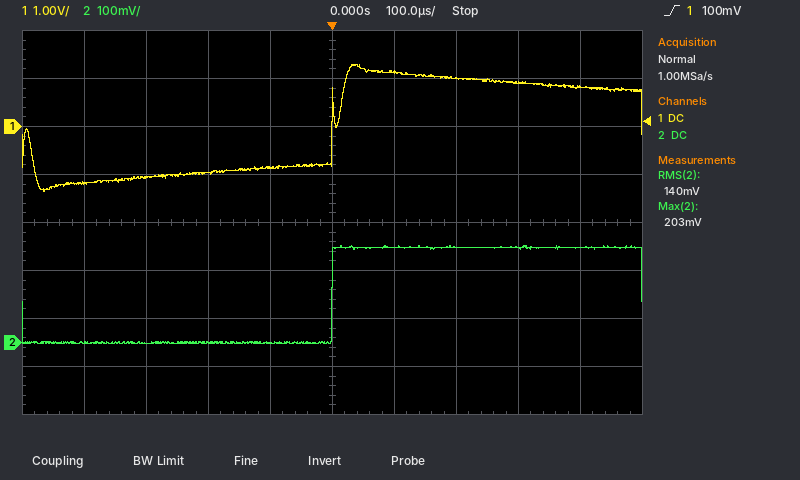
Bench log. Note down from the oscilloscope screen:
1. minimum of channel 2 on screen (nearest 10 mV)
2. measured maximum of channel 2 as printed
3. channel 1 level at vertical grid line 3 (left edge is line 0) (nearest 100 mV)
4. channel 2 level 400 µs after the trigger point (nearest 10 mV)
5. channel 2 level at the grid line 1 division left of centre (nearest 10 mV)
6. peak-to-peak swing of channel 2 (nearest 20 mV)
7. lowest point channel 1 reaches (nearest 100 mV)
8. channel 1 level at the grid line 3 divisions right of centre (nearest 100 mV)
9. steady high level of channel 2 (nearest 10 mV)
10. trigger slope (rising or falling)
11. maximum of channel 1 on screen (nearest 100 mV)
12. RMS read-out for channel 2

0 mV
203 mV
-1.0 V
200 mV
0 mV
200 mV
-1.4 V
900 mV
200 mV
rising
1.3 V
140 mV
